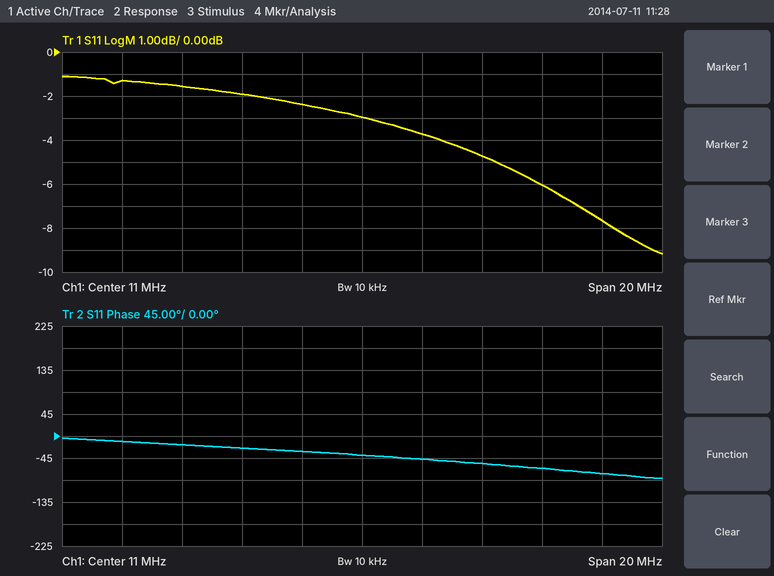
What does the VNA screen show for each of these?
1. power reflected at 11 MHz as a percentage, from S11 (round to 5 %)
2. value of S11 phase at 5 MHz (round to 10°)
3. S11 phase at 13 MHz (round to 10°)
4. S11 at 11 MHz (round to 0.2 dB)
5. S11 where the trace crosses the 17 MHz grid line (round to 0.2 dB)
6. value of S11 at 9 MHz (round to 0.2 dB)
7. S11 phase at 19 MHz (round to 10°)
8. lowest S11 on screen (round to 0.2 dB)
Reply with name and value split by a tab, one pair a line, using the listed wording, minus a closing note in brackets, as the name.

power reflected at 11 MHz as a percentage, from S11	50 %
value of S11 phase at 5 MHz	-20°
S11 phase at 13 MHz	-50°
S11 at 11 MHz	-3.0 dB
S11 where the trace crosses the 17 MHz grid line	-6.0 dB
value of S11 at 9 MHz	-2.4 dB
S11 phase at 19 MHz	-80°
lowest S11 on screen	-9.2 dB
